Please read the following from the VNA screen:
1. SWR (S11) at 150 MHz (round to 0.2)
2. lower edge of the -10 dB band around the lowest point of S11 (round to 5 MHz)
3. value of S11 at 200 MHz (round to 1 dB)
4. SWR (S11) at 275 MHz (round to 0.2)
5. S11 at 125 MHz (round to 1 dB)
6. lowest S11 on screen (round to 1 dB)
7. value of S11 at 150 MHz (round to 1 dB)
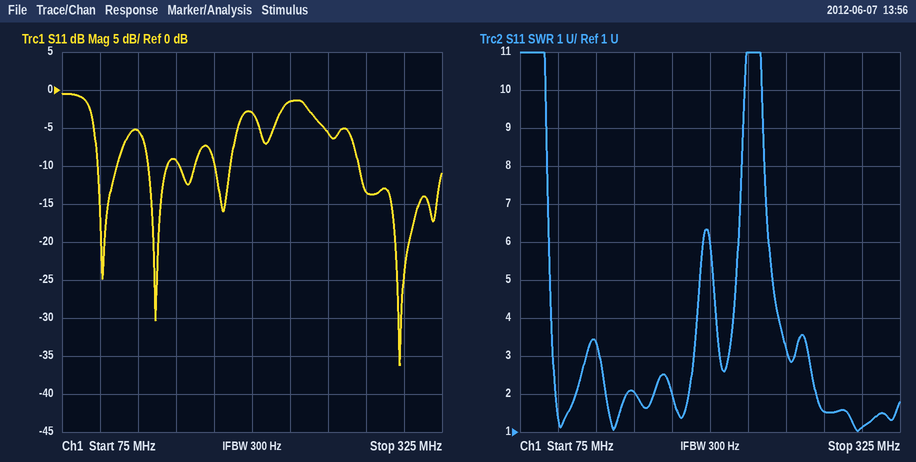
2.0
270 MHz
-3 dB
1.6
-5 dB
-36 dB
-9 dB
